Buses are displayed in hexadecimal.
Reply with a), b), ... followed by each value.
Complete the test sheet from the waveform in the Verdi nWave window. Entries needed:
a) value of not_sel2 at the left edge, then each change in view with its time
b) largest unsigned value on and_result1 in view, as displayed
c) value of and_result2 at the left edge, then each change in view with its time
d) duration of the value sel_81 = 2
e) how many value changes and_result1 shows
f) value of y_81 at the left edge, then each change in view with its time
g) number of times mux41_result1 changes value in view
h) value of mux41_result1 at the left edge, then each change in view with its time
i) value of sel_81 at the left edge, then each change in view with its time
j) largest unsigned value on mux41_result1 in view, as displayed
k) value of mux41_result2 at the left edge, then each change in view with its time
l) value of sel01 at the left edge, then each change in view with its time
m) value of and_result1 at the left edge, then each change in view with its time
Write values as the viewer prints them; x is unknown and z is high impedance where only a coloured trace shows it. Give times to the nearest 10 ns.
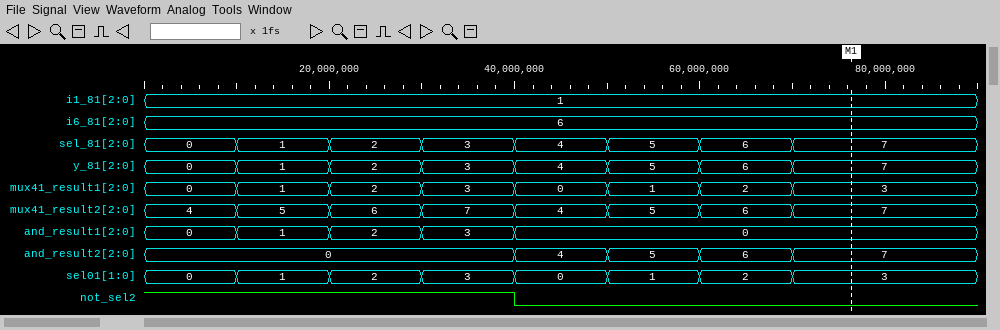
a) 1, 0 at 40 ns
b) 3
c) 0, 4 at 40 ns, 5 at 50 ns, 6 at 60 ns, 7 at 70 ns
d) 10 ns
e) 4
f) 0, 1 at 10 ns, 2 at 20 ns, 3 at 30 ns, 4 at 40 ns, 5 at 50 ns, 6 at 60 ns, 7 at 70 ns
g) 7
h) 0, 1 at 10 ns, 2 at 20 ns, 3 at 30 ns, 0 at 40 ns, 1 at 50 ns, 2 at 60 ns, 3 at 70 ns
i) 0, 1 at 10 ns, 2 at 20 ns, 3 at 30 ns, 4 at 40 ns, 5 at 50 ns, 6 at 60 ns, 7 at 70 ns
j) 3
k) 4, 5 at 10 ns, 6 at 20 ns, 7 at 30 ns, 4 at 40 ns, 5 at 50 ns, 6 at 60 ns, 7 at 70 ns
l) 0, 1 at 10 ns, 2 at 20 ns, 3 at 30 ns, 0 at 40 ns, 1 at 50 ns, 2 at 60 ns, 3 at 70 ns
m) 0, 1 at 10 ns, 2 at 20 ns, 3 at 30 ns, 0 at 40 ns
